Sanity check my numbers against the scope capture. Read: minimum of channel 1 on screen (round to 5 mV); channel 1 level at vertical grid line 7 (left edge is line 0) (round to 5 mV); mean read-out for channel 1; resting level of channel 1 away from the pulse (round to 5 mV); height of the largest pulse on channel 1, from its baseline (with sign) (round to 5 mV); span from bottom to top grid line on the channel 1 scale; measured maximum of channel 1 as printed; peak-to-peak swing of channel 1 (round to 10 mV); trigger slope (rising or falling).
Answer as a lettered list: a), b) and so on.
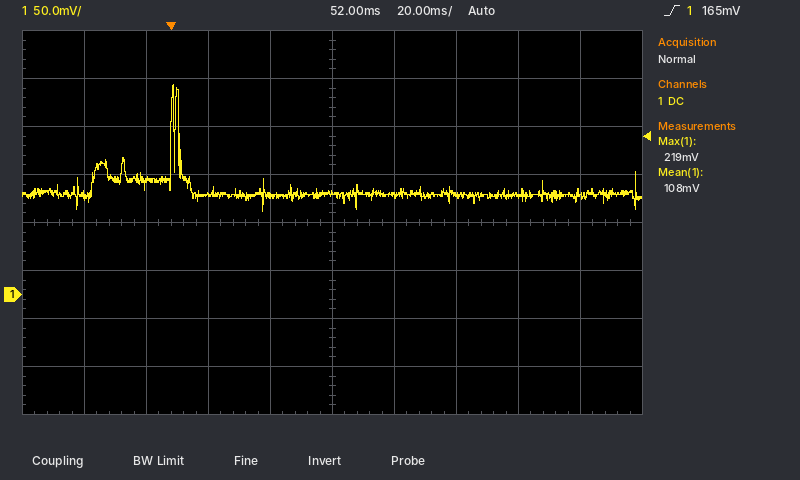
a) 85 mV
b) 105 mV
c) 108 mV
d) 105 mV
e) +115 mV
f) 400 mV
g) 219 mV
h) 130 mV
i) rising
